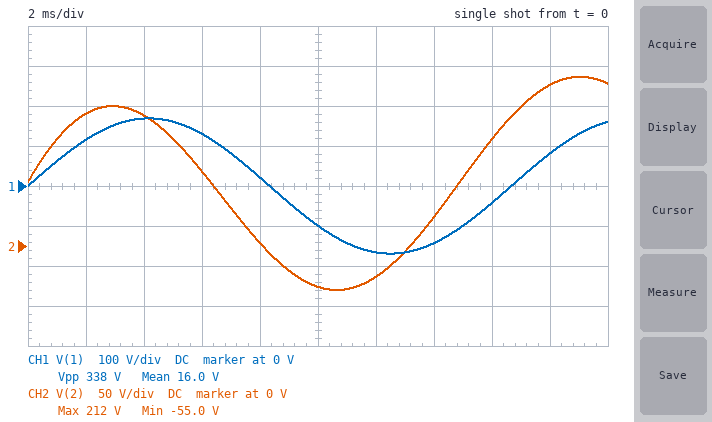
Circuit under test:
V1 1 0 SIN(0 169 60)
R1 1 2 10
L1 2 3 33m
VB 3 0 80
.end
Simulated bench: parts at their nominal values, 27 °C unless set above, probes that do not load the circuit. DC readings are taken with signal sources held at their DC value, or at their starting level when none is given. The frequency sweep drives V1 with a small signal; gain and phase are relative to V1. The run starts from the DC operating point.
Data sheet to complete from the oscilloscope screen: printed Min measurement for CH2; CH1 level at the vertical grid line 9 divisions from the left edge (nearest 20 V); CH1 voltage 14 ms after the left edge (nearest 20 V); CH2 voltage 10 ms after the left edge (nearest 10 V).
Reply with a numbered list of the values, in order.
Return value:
1. -55.0 V
2. 80 V
3. -140 V
4. -50 V
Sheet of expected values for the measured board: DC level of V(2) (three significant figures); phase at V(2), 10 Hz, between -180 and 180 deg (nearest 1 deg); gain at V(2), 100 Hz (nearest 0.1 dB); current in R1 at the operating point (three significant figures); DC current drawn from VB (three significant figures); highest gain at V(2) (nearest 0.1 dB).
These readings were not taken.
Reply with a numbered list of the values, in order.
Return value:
1. 80.0 V
2. 78 deg
3. -0.9 dB
4. 8.00 A
5. 8.00 A
6. 0 dB
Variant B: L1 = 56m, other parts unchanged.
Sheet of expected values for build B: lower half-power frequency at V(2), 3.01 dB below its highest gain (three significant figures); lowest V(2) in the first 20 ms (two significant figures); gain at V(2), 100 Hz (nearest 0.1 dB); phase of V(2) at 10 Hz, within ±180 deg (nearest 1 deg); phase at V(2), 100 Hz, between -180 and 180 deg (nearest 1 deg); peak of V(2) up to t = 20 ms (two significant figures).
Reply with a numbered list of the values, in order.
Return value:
1. 28.4 Hz
2. -81 V
3. -0.3 dB
4. 71 deg
5. 16 deg
6. 230 V
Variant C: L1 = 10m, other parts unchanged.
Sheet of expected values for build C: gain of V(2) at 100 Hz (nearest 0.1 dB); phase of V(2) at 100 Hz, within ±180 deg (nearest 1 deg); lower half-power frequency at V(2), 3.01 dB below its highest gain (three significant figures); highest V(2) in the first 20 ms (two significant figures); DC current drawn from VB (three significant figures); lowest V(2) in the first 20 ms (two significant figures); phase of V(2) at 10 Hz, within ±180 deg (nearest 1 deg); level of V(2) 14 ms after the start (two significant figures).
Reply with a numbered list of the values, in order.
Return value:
1. -5.5 dB
2. 58 deg
3. 159 Hz
4. 140 V
5. 8.00 A
6. 20 V
7. 86 deg
8. 92 V
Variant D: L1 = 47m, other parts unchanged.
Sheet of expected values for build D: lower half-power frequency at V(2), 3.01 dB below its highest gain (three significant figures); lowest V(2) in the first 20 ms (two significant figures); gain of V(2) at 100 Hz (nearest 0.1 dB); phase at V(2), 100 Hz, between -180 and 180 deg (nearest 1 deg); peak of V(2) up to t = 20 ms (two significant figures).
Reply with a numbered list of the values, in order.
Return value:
1. 33.9 Hz
2. -74 V
3. -0.5 dB
4. 19 deg
5. 230 V
